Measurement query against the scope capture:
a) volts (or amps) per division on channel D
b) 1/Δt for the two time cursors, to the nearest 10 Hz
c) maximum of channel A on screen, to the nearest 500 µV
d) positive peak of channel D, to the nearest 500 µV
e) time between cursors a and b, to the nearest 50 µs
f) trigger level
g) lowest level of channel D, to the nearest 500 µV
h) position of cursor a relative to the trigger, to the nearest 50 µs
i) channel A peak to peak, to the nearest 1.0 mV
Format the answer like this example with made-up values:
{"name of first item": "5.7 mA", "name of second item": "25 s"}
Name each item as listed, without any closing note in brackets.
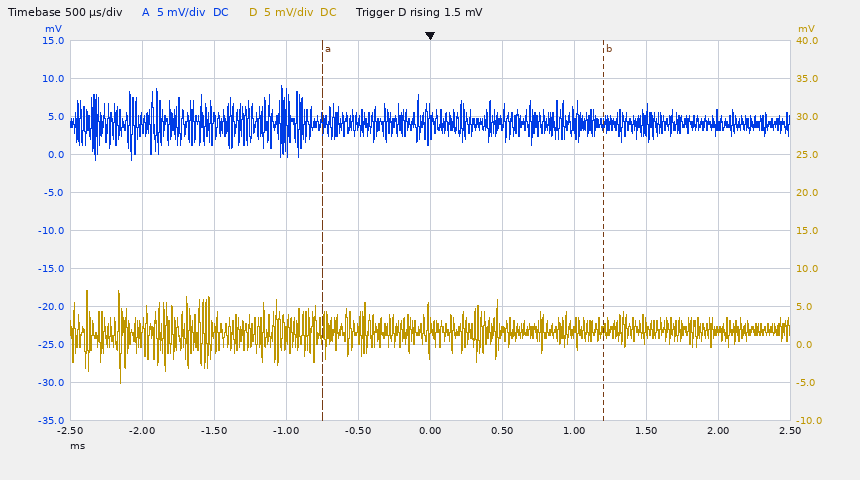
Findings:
{"volts (or amps) per division on channel D": "5 mV", "1/Δt for the two time cursors, to the nearest 10 Hz": "510 Hz", "maximum of channel A on screen, to the nearest 500 µV": "9.0 mV", "positive peak of channel D, to the nearest 500 µV": "7.0 mV", "time between cursors a and b, to the nearest 50 µs": "1.95 ms", "trigger level": "1.5 mV", "lowest level of channel D, to the nearest 500 µV": "-5.0 mV", "position of cursor a relative to the trigger, to the nearest 50 µs": "-750 µs", "channel A peak to peak, to the nearest 1.0 mV": "10.0 mV"}
